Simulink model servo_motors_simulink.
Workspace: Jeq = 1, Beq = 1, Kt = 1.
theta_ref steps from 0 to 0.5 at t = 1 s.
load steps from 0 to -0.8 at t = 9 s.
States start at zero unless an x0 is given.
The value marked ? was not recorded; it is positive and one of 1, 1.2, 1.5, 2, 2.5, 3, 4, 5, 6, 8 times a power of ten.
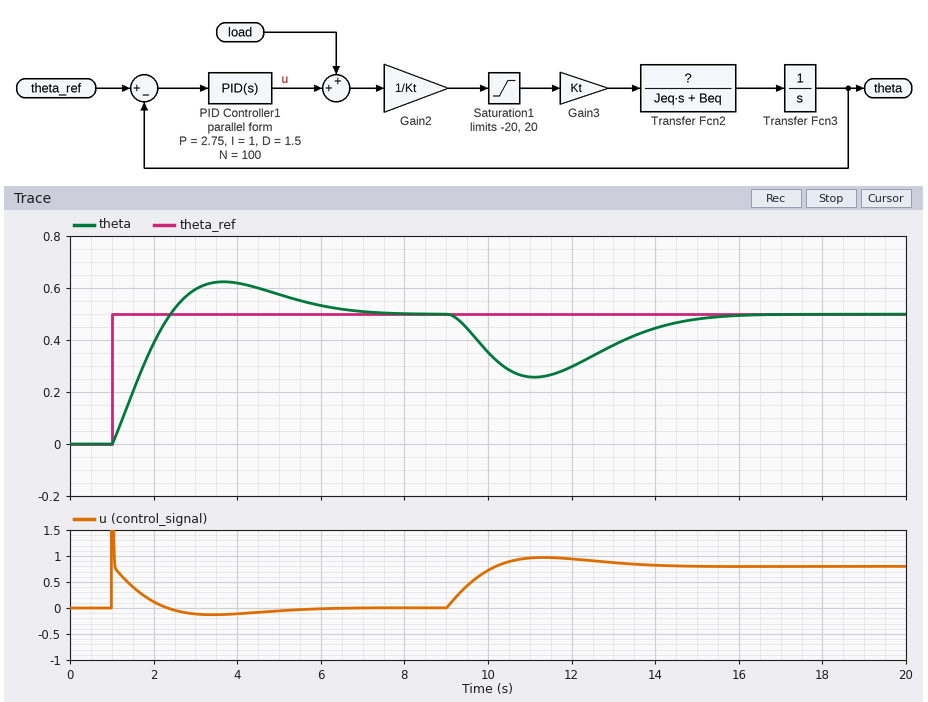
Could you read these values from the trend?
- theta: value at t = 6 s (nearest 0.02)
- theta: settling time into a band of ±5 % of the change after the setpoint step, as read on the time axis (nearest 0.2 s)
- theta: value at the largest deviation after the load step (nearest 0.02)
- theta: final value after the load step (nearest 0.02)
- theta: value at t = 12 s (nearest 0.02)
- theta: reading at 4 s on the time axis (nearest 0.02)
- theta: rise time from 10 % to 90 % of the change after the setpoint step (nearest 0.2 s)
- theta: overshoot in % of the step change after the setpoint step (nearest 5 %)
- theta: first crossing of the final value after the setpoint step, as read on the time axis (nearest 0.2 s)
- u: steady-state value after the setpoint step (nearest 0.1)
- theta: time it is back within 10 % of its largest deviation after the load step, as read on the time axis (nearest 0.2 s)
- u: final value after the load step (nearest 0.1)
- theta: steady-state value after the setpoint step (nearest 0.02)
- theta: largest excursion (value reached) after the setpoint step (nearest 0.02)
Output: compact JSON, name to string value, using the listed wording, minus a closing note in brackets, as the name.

{"theta: value at t = 6 s": "0.54", "theta: settling time into a band of ±5 % of the change after the setpoint step, as read on the time axis": "6.2 s", "theta: value at the largest deviation after the load step": "0.26", "theta: final value after the load step": "0.50", "theta: value at t = 12 s": "0.30", "theta: reading at 4 s on the time axis": "0.62", "theta: rise time from 10 % to 90 % of the change after the setpoint step": "1.0 s", "theta: overshoot in % of the step change after the setpoint step": "25 %", "theta: first crossing of the final value after the setpoint step, as read on the time axis": "2.4 s", "u: steady-state value after the setpoint step": "0.0", "theta: time it is back within 10 % of its largest deviation after the load step, as read on the time axis": "14.8 s", "u: final value after the load step": "0.8", "theta: steady-state value after the setpoint step": "0.50", "theta: largest excursion (value reached) after the setpoint step": "0.62"}
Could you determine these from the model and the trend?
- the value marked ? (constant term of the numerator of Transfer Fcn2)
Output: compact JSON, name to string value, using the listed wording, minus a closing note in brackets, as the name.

{"the value marked ?": "0.8"}
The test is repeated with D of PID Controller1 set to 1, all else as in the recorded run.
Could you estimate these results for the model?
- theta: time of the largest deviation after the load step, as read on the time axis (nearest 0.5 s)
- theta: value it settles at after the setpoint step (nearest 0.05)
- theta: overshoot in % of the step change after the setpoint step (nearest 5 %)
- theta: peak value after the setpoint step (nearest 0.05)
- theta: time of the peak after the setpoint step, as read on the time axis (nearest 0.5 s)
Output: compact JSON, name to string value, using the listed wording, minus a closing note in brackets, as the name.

{"theta: time of the largest deviation after the load step, as read on the time axis": "11.0 s", "theta: value it settles at after the setpoint step": "0.50", "theta: overshoot in % of the step change after the setpoint step": "30 %", "theta: peak value after the setpoint step": "0.65", "theta: time of the peak after the setpoint step, as read on the time axis": "3.5 s"}
